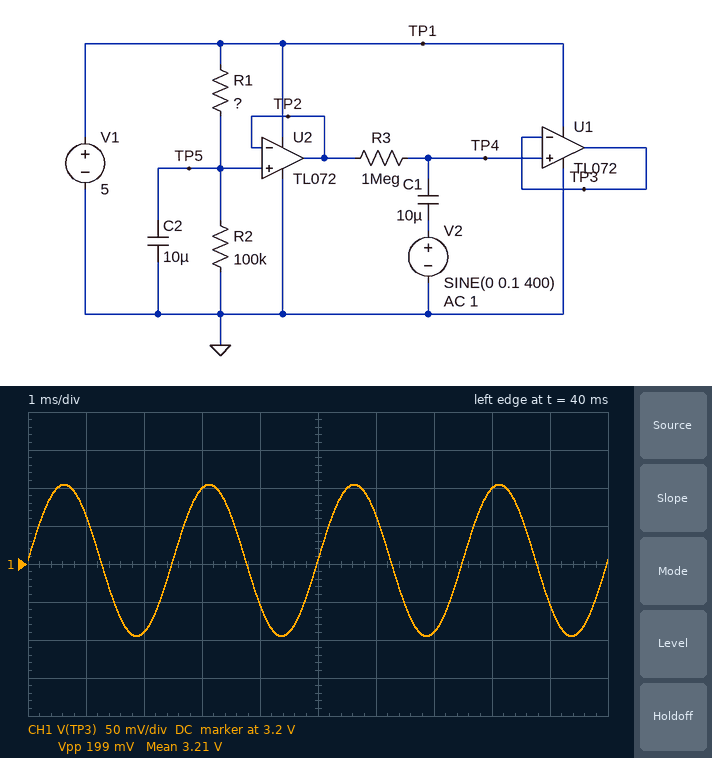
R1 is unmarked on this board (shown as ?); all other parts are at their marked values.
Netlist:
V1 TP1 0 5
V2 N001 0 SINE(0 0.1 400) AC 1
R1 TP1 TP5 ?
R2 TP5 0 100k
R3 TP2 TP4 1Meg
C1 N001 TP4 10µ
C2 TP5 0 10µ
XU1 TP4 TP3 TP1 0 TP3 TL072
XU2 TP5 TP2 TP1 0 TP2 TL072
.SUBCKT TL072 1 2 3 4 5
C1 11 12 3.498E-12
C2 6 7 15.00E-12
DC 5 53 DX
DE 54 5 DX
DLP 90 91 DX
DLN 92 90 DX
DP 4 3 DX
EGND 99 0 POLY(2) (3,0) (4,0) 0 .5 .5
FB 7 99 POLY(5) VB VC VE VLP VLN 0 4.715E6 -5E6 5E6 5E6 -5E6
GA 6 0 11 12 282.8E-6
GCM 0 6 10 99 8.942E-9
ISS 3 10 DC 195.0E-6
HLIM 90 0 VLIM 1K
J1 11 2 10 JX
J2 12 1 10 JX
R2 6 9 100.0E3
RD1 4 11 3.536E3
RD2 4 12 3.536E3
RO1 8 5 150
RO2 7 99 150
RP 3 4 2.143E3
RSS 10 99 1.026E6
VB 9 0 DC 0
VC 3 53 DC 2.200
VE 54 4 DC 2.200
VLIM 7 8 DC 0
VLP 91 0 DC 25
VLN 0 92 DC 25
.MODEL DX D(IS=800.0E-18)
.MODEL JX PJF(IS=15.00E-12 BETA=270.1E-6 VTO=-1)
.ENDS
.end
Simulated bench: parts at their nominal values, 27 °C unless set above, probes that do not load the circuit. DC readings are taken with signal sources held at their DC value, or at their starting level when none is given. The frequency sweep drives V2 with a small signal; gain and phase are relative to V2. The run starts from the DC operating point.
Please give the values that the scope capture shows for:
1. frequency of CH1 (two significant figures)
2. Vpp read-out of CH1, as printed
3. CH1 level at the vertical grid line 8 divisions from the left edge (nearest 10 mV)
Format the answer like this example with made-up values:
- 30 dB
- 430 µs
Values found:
- 400 Hz
- 199 mV
- 3.30 V
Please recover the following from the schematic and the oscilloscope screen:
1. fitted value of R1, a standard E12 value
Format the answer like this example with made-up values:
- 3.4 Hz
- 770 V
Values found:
- 56 kΩ
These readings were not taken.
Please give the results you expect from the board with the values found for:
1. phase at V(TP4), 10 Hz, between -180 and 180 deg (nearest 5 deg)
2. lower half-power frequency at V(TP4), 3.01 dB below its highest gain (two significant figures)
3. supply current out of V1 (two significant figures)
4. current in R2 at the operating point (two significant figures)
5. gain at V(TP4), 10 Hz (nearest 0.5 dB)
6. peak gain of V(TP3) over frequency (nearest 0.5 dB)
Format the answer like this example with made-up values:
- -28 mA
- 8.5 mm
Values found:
- 0 deg
- 16 mHz
- 5.1 mA
- 32 µA
- 0 dB
- 0 dB
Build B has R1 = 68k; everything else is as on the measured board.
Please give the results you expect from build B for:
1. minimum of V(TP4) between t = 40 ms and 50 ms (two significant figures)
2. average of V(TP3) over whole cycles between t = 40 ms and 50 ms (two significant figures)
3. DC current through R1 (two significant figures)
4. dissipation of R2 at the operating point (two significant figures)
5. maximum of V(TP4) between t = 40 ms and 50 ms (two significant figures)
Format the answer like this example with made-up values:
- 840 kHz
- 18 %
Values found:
- 2.9 V
- 3.0 V
- 30 µA
- 89 µW
- 3.1 V
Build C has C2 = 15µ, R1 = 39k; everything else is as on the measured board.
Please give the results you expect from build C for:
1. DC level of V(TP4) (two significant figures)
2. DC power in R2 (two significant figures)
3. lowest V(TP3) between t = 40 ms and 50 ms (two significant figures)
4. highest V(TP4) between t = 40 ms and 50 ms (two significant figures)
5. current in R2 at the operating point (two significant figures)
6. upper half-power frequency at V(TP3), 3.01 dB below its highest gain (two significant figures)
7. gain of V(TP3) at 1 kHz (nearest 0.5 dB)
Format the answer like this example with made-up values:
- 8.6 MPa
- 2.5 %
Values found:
- 3.4 V
- 130 µW
- 3.3 V
- 3.5 V
- 36 µA
- 180 kHz
- -7.5 dB
